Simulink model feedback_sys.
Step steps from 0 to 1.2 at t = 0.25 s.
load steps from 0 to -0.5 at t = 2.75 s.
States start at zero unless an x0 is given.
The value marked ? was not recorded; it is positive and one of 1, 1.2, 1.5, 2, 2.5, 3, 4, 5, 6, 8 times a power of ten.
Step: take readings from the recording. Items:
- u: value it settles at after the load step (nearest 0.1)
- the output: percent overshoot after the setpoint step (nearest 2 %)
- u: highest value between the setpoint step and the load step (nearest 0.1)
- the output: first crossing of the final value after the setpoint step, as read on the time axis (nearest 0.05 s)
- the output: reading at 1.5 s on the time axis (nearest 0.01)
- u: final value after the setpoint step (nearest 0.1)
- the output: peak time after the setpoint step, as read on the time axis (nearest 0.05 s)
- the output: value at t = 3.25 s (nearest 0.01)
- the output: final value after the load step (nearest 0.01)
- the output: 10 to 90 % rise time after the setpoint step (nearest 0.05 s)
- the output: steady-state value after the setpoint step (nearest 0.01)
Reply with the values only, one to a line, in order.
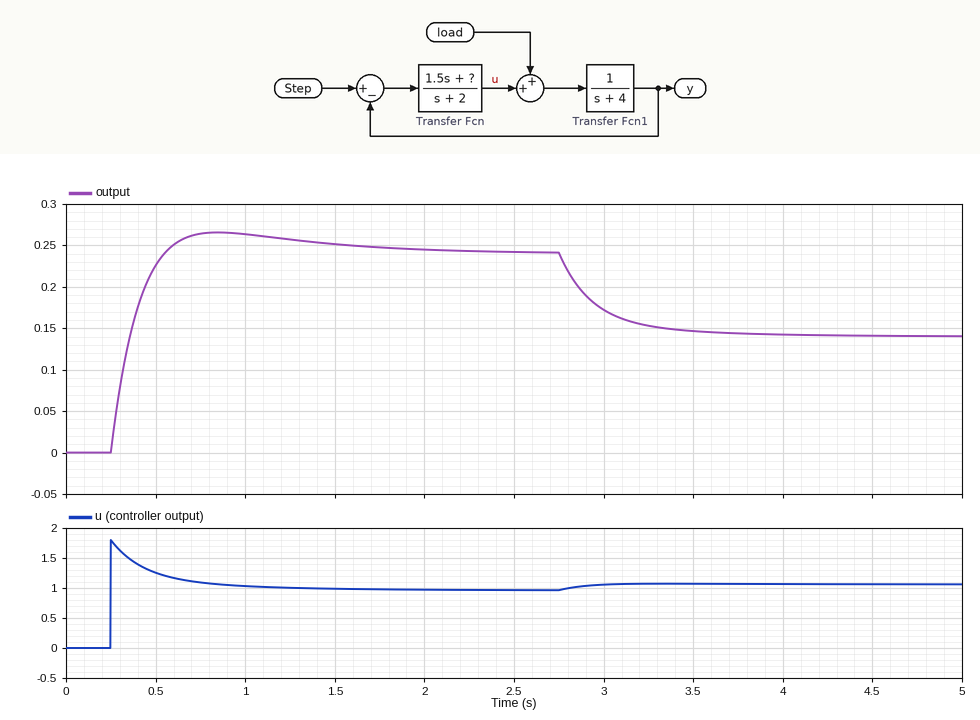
1.1
10 %
1.8
0.55 s
0.25
1.0
0.85 s
0.15
0.14
0.20 s
0.24
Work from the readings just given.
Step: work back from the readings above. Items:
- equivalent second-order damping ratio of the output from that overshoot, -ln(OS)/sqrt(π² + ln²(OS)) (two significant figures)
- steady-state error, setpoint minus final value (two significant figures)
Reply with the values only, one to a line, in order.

0.59
0.96
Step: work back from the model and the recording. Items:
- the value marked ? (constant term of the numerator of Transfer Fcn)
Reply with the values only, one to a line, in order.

2
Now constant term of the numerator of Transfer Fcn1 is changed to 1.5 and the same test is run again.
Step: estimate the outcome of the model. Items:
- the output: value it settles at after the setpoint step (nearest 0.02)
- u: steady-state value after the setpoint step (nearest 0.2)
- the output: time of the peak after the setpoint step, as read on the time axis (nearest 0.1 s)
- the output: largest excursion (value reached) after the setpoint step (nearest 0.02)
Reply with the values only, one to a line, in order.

0.32
0.8
0.8 s
0.36
